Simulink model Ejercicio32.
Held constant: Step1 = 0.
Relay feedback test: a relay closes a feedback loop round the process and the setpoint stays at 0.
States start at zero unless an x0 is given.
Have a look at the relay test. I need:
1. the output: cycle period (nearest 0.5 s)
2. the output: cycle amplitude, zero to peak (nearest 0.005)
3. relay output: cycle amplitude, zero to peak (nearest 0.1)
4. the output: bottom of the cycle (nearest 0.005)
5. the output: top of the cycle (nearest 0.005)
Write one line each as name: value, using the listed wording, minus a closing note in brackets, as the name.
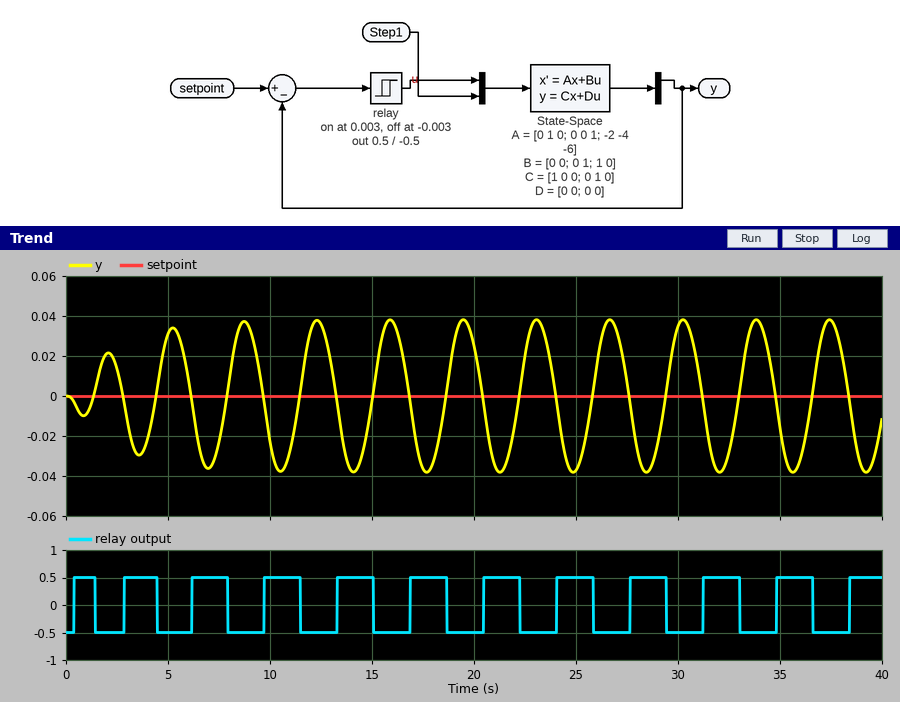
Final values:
the output: cycle period: 3.5 s
the output: cycle amplitude, zero to peak: 0.040
relay output: cycle amplitude, zero to peak: 0.5
the output: bottom of the cycle: -0.040
the output: top of the cycle: 0.040
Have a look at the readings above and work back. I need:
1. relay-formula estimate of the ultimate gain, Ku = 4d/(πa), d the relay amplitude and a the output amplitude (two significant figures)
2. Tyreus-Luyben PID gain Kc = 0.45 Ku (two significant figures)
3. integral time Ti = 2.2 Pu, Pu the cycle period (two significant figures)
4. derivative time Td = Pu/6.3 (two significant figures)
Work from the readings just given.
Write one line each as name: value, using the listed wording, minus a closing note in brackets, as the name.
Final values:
relay-formula estimate of the ultimate gain, Ku = 4d/(πa), d the relay amplitude and a the output amplitude: 16
Tyreus-Luyben PID gain Kc = 0.45 Ku: 7.2
integral time Ti = 2.2 Pu, Pu the cycle period: 7.7 s
derivative time Td = Pu/6.3: 0.56 s
